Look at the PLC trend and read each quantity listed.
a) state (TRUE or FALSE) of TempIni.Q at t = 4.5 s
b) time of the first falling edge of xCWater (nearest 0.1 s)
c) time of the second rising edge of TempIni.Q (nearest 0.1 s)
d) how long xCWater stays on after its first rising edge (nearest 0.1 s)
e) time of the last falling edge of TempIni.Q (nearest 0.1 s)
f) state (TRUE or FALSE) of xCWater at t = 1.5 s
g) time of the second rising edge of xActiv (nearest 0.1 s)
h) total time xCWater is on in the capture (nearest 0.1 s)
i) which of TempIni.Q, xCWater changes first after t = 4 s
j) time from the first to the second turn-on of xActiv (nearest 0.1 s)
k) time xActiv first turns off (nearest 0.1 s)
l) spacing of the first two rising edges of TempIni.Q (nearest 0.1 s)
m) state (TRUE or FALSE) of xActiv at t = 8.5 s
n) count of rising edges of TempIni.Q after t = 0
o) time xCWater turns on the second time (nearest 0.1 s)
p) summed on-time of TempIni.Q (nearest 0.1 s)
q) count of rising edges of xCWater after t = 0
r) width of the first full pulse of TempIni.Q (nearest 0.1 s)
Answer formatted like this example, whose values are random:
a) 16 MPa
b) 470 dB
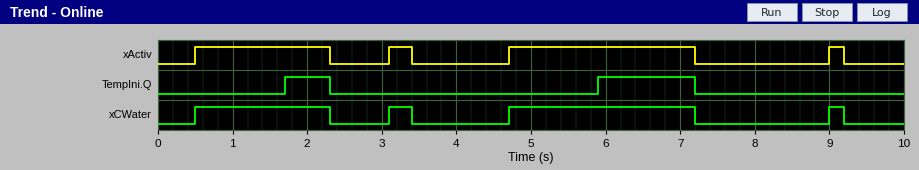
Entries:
a) FALSE
b) 2.3 s
c) 5.9 s
d) 1.8 s
e) 7.2 s
f) TRUE
g) 3.1 s
h) 4.8 s
i) xCWater
j) 2.6 s
k) 2.3 s
l) 4.2 s
m) FALSE
n) 2
o) 3.1 s
p) 1.9 s
q) 4
r) 0.6 s
